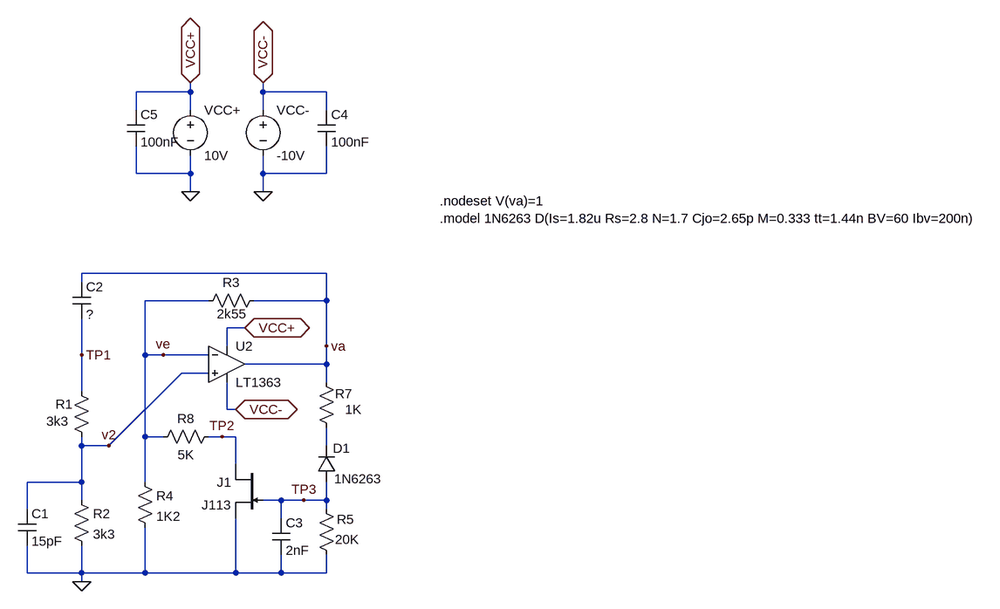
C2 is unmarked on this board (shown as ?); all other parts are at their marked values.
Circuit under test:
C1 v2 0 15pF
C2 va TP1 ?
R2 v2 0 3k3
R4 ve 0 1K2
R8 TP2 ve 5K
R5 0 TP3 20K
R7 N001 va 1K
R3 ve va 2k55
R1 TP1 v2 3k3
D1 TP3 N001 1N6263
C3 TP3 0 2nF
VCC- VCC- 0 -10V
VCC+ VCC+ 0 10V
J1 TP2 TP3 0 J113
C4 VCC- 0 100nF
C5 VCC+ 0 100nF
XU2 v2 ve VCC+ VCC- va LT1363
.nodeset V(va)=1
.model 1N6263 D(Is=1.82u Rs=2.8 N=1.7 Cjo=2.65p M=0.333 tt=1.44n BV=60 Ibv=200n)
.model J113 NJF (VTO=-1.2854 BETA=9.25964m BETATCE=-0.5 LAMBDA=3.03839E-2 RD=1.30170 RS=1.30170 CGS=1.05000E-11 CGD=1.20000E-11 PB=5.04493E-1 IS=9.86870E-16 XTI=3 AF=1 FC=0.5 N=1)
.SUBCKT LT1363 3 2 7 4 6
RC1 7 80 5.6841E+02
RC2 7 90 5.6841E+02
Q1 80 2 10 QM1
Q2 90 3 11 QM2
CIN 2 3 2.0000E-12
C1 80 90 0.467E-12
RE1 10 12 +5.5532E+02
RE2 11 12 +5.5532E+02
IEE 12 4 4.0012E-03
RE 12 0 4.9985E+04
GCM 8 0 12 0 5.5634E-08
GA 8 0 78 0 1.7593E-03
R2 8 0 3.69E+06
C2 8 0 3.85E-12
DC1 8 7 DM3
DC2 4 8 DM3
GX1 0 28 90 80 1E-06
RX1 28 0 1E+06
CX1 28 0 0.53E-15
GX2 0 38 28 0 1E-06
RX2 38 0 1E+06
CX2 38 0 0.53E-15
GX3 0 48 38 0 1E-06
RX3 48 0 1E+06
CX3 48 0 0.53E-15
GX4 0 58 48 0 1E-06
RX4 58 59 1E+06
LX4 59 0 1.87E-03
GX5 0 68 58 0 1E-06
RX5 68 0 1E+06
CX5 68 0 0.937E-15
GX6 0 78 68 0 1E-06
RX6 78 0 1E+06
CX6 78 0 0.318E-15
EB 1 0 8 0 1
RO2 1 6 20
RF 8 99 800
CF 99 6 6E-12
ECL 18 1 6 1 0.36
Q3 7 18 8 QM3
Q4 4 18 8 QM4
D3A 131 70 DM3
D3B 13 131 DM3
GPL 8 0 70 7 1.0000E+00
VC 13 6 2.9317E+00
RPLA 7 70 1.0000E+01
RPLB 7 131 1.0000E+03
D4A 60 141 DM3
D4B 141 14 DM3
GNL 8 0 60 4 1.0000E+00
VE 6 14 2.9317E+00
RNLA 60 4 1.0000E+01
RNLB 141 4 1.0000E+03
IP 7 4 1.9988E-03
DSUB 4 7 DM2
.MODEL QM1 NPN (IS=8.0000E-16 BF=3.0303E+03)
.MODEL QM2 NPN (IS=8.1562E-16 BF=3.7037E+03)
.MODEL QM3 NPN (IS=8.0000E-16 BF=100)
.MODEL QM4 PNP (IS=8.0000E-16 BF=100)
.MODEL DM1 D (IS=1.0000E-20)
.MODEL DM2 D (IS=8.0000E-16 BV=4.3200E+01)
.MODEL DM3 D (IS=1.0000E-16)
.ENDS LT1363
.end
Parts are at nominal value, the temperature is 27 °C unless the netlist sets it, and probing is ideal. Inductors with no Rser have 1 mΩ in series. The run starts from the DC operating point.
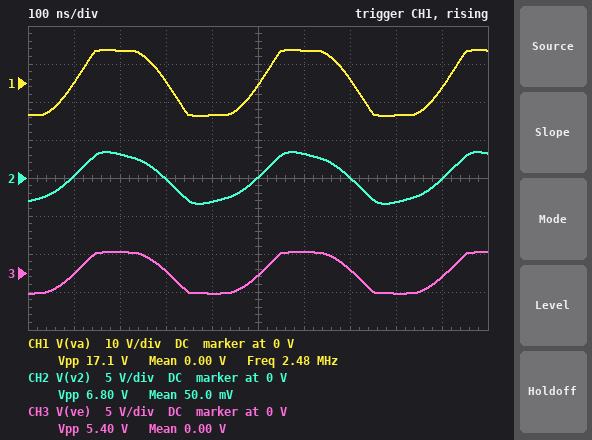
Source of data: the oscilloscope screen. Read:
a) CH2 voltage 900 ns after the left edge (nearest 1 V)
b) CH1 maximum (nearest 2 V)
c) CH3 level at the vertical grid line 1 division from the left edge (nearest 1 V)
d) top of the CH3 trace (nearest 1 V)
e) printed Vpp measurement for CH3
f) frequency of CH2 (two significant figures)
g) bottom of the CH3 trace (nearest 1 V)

0 V
8 V
0 V
3 V
5.40 V
2.5 MHz
-3 V
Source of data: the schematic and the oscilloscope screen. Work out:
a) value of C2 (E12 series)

18 pF
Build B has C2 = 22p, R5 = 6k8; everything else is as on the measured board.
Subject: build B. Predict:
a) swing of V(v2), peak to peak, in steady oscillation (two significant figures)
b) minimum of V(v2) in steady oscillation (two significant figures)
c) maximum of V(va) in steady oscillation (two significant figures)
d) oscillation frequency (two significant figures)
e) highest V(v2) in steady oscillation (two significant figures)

7.4 V
-3.7 V
8.6 V
2.2 MHz
3.7 V
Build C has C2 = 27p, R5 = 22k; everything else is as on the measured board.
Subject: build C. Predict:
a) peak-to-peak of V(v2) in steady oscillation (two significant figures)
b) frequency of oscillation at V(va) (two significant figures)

7.9 V
1.9 MHz
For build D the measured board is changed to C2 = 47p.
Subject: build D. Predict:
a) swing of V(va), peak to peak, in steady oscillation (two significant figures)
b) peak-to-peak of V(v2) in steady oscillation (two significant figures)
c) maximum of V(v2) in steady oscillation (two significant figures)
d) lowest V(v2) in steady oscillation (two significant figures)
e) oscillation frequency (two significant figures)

17 V
9.1 V
4.5 V
-4.5 V
1.3 MHz
